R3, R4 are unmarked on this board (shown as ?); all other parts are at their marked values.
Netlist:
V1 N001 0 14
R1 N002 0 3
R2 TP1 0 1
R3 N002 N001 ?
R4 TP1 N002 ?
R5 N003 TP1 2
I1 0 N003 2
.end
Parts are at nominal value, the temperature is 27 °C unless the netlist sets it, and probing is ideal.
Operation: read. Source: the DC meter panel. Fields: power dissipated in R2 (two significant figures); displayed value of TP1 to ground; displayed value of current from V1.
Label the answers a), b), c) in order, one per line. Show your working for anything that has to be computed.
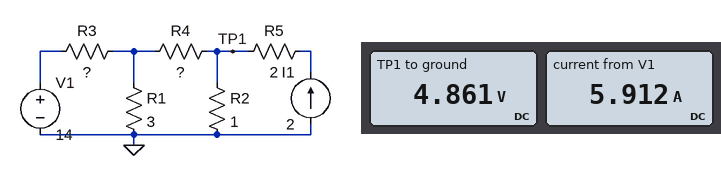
a) (4.861 V)^2 / 1 Ω = 24 W
b) 4.861 V
c) 5.912 A
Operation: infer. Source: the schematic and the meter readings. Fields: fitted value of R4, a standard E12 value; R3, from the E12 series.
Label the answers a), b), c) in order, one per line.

a) 1.5 Ω
b) 0.82 Ω
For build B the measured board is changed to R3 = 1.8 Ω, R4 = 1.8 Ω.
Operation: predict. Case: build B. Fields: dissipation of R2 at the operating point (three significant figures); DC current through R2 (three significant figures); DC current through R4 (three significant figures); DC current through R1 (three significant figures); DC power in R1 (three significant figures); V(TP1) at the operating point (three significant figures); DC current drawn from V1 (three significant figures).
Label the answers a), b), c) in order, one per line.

a) 13.8 W
b) 3.72 A
c) 1.72 A
d) 2.27 A
e) 15.5 W
f) 3.72 V
g) 3.99 A
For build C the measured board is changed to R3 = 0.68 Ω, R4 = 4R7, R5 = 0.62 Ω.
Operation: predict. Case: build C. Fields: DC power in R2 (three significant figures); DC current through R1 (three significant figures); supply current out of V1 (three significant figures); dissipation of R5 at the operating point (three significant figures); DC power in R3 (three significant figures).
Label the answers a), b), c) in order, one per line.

a) 12.3 W
b) 3.53 A
c) 5.03 A
d) 2.48 W
e) 17.2 W
